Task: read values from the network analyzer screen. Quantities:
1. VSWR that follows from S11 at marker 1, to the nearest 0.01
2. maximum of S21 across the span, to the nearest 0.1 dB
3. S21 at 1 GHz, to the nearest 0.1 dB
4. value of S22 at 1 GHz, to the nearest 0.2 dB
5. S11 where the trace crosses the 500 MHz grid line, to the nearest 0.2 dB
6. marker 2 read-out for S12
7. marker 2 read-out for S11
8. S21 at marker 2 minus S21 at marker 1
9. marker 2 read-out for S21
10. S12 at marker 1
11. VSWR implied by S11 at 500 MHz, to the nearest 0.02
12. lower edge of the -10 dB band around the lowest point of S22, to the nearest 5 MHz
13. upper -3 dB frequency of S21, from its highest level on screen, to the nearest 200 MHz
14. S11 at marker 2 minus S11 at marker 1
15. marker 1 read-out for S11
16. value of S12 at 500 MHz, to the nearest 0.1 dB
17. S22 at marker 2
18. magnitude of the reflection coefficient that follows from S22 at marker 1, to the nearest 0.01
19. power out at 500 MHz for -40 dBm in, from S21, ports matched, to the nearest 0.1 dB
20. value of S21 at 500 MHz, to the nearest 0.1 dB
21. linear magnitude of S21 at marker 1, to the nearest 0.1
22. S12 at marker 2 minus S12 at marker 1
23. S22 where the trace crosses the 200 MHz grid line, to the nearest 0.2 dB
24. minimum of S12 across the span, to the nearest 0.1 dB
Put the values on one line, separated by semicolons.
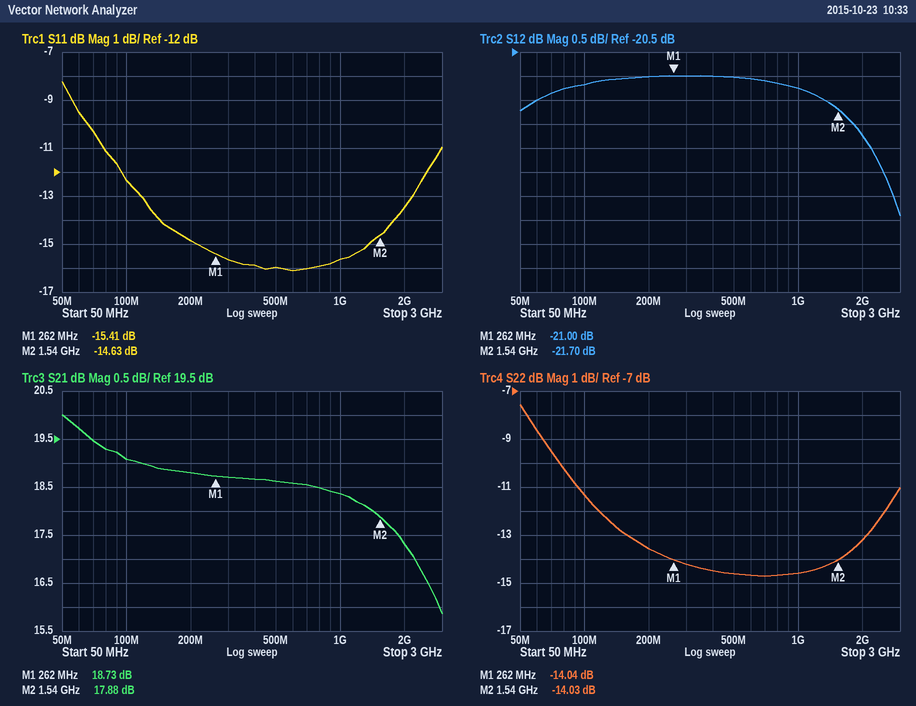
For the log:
1.41; 20.0 dB; 18.4 dB; -14.6 dB; -16.0 dB; -21.70 dB; -14.63 dB; -0.85 dB; 17.88 dB; -21.00 dB; 1.38; 75 MHz; 2.2 GHz; 0.78 dB; -15.41 dB; -21.0 dB; -14.03 dB; 0.20; -21.4 dBm; 18.6 dB; 8.6; -0.70 dB; -13.6 dB; -23.9 dB
